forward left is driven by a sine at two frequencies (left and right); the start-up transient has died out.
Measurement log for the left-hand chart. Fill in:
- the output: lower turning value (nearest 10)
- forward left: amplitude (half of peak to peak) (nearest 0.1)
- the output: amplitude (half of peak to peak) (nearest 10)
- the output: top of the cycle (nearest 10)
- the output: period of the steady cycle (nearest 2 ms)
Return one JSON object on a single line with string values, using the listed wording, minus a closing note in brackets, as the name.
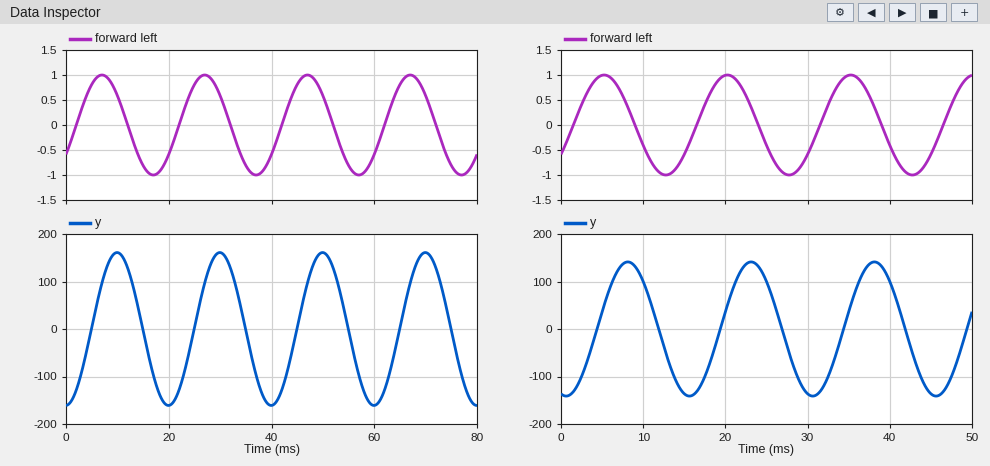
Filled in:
{"the output: lower turning value": "-160", "forward left: amplitude (half of peak to peak)": "1.0", "the output: amplitude (half of peak to peak)": "160", "the output: top of the cycle": "160", "the output: period of the steady cycle": "20 ms"}
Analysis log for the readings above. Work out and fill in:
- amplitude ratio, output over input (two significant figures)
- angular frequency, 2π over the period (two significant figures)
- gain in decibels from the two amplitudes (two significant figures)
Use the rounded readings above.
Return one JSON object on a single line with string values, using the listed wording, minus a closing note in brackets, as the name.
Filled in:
{"amplitude ratio, output over input": "160", "angular frequency, 2π over the period": "0.31 rad/ms", "gain in decibels from the two amplitudes": "44 dB"}
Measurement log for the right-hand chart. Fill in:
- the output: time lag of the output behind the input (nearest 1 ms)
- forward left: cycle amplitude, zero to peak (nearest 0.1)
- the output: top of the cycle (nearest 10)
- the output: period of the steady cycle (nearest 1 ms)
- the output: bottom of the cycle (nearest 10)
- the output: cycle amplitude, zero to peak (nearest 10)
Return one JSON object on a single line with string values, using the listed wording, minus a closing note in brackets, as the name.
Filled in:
{"the output: time lag of the output behind the input": "3 ms", "forward left: cycle amplitude, zero to peak": "1.0", "the output: top of the cycle": "140", "the output: period of the steady cycle": "15 ms", "the output: bottom of the cycle": "-140", "the output: cycle amplitude, zero to peak": "140"}
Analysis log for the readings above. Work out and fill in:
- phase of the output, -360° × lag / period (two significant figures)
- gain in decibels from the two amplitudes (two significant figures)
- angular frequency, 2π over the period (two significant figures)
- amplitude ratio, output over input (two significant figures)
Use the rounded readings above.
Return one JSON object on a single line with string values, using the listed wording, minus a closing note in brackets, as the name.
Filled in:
{"phase of the output, -360° × lag / period": "-72°", "gain in decibels from the two amplitudes": "43 dB", "angular frequency, 2π over the period": "0.42 rad/ms", "amplitude ratio, output over input": "140"}
